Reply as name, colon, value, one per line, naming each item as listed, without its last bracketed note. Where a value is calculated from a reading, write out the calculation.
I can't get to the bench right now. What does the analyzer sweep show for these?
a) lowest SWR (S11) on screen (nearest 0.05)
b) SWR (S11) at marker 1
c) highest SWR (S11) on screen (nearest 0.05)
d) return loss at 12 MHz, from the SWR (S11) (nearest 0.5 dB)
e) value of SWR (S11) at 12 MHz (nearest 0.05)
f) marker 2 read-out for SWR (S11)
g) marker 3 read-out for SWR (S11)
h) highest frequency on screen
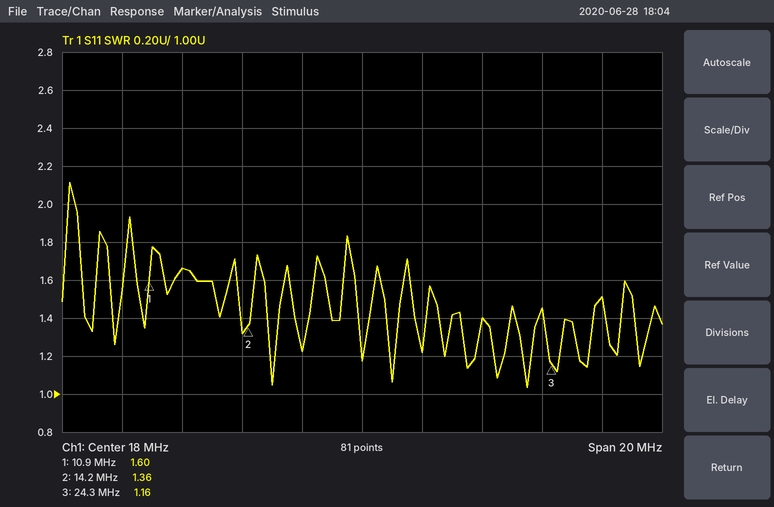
lowest SWR (S11) on screen: 1.05
SWR (S11) at marker 1: 1.60
highest SWR (S11) on screen: 2.10
return loss at 12 MHz, from the SWR (S11): −20 log10((1.65 − 1)/(1.65 + 1)) ≈ 12.2 dB, so 12.0 dB to the nearest 0.5 dB
value of SWR (S11) at 12 MHz: 1.65
marker 2 read-out for SWR: 1.36
marker 3 read-out for SWR: 1.16
highest frequency on screen: 28 MHz
